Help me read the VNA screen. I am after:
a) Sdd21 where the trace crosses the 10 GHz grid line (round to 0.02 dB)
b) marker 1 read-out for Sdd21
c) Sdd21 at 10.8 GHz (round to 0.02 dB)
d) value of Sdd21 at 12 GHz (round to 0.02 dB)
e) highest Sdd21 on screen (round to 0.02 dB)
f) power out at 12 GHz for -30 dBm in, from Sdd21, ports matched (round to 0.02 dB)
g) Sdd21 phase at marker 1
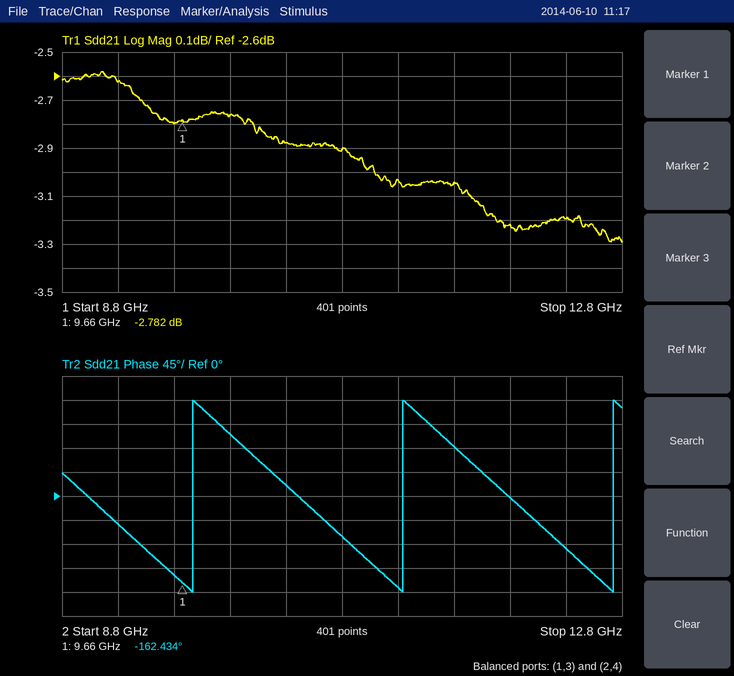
-2.76 dB
-2.782 dB
-2.90 dB
-3.22 dB
-2.58 dB
-33.22 dBm
-162.434°
